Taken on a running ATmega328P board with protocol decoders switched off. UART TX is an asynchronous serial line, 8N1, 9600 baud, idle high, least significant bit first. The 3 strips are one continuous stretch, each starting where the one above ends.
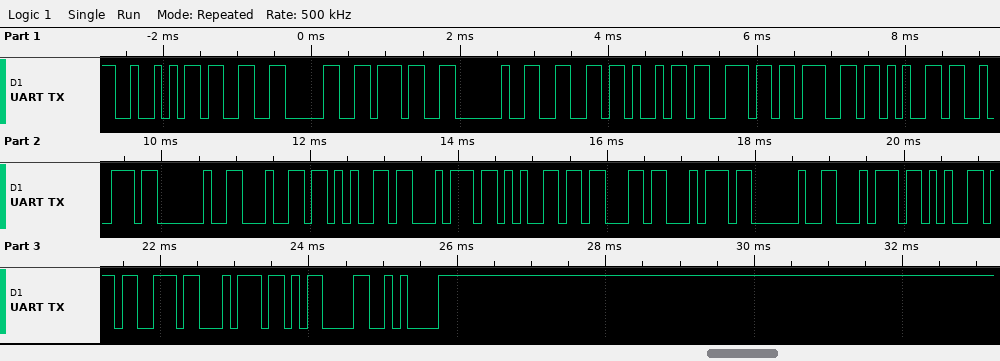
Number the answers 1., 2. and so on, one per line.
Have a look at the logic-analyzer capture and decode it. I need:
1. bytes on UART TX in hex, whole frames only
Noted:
1. 52 33 30 37 20 66 69 6E 67 65 72 20 64 65 74 65 63 74 20 74 65 73 74 0D 0A
